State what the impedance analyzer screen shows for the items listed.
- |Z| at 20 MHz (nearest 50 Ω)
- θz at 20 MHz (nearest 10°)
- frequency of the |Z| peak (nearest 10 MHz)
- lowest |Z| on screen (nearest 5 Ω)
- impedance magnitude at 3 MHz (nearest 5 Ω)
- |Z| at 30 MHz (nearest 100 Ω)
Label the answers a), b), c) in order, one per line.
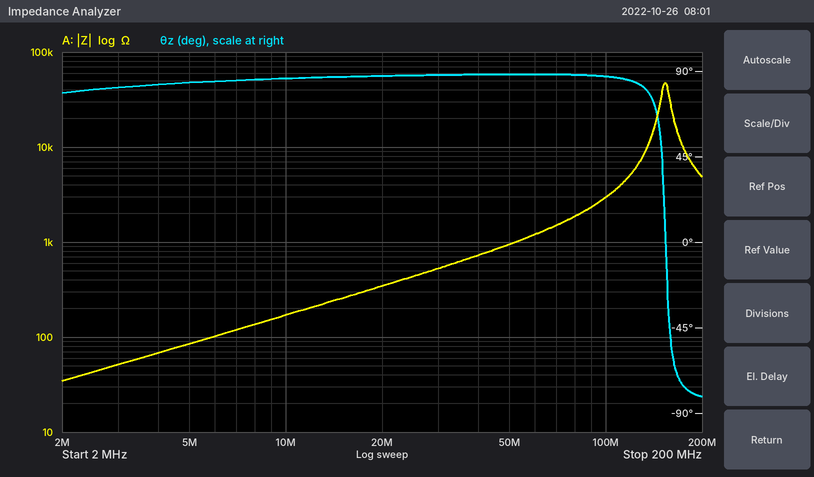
a) 350 Ω
b) 90°
c) 150 MHz
d) 35 Ω
e) 50 Ω
f) 500 Ω
